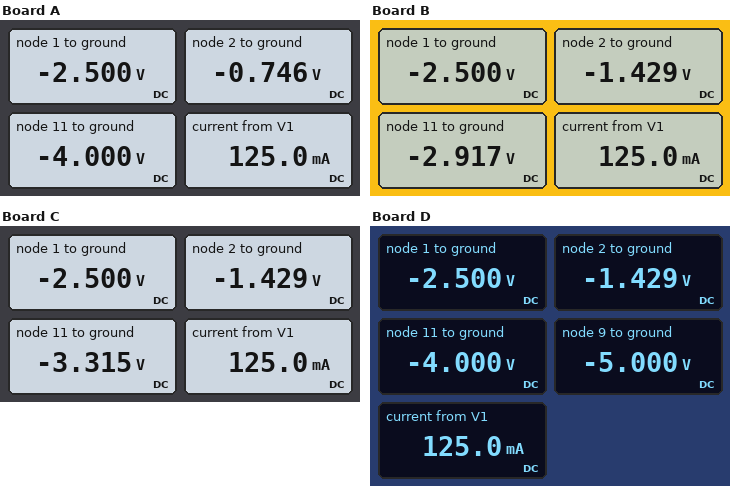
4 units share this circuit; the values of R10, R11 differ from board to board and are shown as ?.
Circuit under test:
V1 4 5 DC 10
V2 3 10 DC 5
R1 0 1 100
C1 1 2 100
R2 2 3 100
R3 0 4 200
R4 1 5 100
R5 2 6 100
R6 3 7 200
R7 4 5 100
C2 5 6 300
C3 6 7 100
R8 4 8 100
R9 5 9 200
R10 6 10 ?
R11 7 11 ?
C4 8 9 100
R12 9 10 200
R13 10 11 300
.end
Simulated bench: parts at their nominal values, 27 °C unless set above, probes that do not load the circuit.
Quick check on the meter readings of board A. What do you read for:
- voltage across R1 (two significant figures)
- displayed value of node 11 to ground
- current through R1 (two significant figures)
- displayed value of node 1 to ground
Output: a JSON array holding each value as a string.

["2.5 V", "-4.000 V", "25 mA", "-2.500 V"]
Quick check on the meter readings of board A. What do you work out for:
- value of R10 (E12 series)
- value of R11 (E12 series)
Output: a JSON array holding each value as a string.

["470 Ω", "1 kΩ"]
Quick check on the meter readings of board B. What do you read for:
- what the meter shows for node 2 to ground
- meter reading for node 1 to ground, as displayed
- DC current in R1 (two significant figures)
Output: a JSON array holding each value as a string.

["-1.429 V", "-2.500 V", "25 mA"]
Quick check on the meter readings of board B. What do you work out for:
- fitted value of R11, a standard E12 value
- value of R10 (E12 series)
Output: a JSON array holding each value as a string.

["220 Ω", "150 Ω"]
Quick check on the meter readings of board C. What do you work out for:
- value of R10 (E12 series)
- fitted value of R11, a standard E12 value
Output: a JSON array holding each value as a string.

["150 Ω", "390 Ω"]
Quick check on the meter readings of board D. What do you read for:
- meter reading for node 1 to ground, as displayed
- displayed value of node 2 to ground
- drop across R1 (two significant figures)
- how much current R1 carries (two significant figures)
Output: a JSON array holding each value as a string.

["-2.500 V", "-1.429 V", "2.5 V", "25 mA"]
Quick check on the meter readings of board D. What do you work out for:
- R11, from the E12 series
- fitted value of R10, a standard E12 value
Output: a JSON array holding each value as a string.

["1 kΩ", "150 Ω"]
